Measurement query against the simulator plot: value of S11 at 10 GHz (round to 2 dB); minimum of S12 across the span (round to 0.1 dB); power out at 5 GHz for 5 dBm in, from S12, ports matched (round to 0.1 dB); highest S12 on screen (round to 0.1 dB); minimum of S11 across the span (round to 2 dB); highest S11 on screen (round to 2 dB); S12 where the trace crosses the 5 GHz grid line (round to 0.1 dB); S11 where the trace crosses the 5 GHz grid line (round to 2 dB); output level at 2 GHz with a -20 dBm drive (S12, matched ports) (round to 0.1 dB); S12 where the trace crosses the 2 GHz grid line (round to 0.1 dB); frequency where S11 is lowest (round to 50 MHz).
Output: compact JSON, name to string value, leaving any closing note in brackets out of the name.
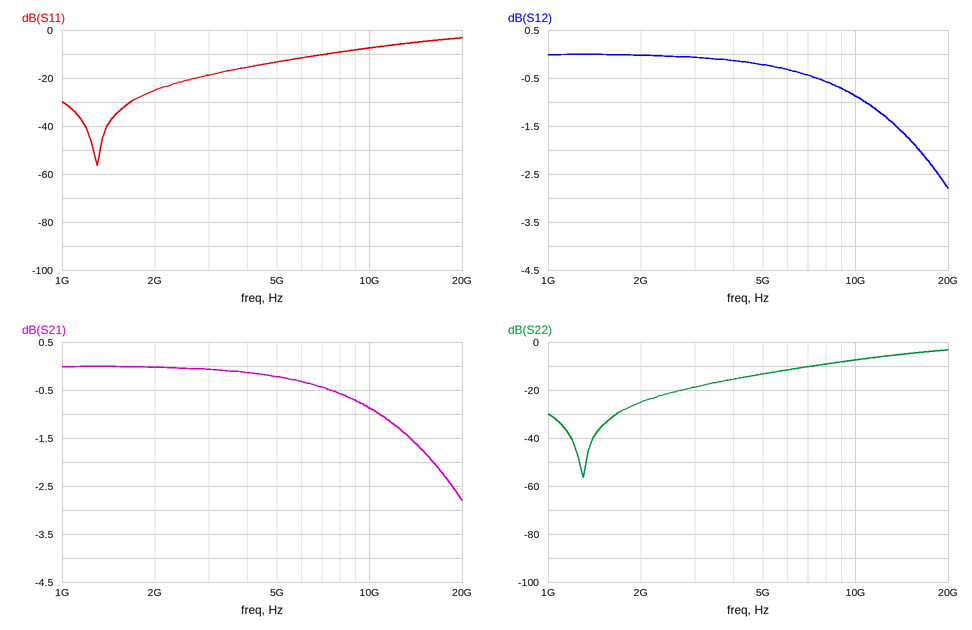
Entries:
{"value of S11 at 10 GHz": "-8 dB", "minimum of S12 across the span": "-2.8 dB", "power out at 5 GHz for 5 dBm in, from S12, ports matched": "4.8 dBm", "highest S12 on screen": "0.0 dB", "minimum of S11 across the span": "-56 dB", "highest S11 on screen": "-4 dB", "S12 where the trace crosses the 5 GHz grid line": "-0.2 dB", "S11 where the trace crosses the 5 GHz grid line": "-14 dB", "output level at 2 GHz with a -20 dBm drive (S12, matched ports)": "-20.0 dBm", "S12 where the trace crosses the 2 GHz grid line": "0.0 dB", "frequency where S11 is lowest": "1.30 GHz"}
